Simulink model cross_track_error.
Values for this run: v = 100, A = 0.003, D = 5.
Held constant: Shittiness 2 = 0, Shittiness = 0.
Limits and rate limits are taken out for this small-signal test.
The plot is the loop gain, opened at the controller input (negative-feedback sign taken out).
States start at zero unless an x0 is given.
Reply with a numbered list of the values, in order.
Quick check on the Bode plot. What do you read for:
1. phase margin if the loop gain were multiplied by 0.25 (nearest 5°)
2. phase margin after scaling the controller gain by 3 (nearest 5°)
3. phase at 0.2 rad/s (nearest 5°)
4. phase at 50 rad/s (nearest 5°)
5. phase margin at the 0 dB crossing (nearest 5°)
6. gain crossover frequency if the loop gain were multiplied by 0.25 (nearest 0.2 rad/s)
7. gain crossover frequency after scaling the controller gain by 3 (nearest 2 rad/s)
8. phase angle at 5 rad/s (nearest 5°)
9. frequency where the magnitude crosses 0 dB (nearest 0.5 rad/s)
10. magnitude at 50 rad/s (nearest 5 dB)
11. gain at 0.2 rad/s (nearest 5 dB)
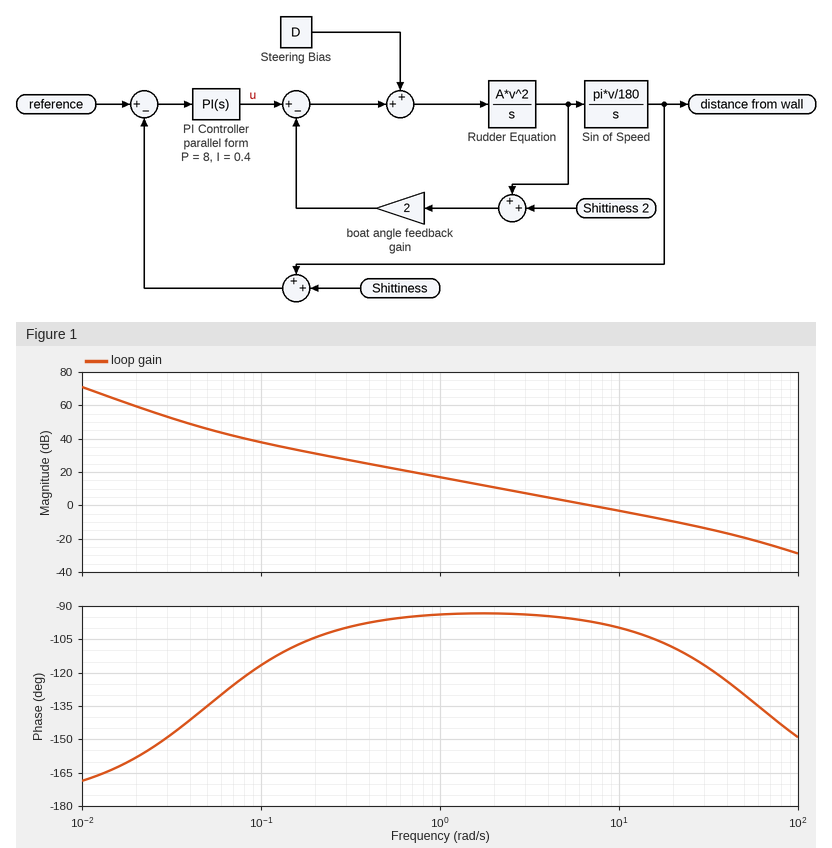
1. 85°
2. 70°
3. -105°
4. -130°
5. 85°
6. 1.8 rad/s
7. 20 rad/s
8. -95°
9. 7.0 rad/s
10. -20 dB
11. 30 dB
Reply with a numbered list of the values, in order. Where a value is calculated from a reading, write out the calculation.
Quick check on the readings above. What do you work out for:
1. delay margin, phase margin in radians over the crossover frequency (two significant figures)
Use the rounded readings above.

1. 85 × π / 180 / 7 = 0.21 s
